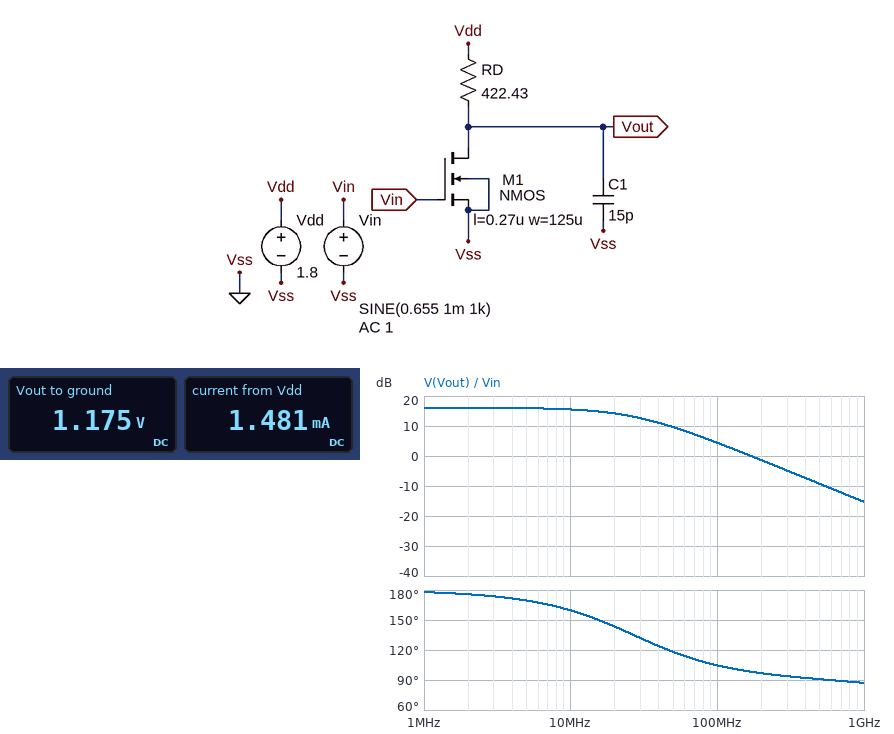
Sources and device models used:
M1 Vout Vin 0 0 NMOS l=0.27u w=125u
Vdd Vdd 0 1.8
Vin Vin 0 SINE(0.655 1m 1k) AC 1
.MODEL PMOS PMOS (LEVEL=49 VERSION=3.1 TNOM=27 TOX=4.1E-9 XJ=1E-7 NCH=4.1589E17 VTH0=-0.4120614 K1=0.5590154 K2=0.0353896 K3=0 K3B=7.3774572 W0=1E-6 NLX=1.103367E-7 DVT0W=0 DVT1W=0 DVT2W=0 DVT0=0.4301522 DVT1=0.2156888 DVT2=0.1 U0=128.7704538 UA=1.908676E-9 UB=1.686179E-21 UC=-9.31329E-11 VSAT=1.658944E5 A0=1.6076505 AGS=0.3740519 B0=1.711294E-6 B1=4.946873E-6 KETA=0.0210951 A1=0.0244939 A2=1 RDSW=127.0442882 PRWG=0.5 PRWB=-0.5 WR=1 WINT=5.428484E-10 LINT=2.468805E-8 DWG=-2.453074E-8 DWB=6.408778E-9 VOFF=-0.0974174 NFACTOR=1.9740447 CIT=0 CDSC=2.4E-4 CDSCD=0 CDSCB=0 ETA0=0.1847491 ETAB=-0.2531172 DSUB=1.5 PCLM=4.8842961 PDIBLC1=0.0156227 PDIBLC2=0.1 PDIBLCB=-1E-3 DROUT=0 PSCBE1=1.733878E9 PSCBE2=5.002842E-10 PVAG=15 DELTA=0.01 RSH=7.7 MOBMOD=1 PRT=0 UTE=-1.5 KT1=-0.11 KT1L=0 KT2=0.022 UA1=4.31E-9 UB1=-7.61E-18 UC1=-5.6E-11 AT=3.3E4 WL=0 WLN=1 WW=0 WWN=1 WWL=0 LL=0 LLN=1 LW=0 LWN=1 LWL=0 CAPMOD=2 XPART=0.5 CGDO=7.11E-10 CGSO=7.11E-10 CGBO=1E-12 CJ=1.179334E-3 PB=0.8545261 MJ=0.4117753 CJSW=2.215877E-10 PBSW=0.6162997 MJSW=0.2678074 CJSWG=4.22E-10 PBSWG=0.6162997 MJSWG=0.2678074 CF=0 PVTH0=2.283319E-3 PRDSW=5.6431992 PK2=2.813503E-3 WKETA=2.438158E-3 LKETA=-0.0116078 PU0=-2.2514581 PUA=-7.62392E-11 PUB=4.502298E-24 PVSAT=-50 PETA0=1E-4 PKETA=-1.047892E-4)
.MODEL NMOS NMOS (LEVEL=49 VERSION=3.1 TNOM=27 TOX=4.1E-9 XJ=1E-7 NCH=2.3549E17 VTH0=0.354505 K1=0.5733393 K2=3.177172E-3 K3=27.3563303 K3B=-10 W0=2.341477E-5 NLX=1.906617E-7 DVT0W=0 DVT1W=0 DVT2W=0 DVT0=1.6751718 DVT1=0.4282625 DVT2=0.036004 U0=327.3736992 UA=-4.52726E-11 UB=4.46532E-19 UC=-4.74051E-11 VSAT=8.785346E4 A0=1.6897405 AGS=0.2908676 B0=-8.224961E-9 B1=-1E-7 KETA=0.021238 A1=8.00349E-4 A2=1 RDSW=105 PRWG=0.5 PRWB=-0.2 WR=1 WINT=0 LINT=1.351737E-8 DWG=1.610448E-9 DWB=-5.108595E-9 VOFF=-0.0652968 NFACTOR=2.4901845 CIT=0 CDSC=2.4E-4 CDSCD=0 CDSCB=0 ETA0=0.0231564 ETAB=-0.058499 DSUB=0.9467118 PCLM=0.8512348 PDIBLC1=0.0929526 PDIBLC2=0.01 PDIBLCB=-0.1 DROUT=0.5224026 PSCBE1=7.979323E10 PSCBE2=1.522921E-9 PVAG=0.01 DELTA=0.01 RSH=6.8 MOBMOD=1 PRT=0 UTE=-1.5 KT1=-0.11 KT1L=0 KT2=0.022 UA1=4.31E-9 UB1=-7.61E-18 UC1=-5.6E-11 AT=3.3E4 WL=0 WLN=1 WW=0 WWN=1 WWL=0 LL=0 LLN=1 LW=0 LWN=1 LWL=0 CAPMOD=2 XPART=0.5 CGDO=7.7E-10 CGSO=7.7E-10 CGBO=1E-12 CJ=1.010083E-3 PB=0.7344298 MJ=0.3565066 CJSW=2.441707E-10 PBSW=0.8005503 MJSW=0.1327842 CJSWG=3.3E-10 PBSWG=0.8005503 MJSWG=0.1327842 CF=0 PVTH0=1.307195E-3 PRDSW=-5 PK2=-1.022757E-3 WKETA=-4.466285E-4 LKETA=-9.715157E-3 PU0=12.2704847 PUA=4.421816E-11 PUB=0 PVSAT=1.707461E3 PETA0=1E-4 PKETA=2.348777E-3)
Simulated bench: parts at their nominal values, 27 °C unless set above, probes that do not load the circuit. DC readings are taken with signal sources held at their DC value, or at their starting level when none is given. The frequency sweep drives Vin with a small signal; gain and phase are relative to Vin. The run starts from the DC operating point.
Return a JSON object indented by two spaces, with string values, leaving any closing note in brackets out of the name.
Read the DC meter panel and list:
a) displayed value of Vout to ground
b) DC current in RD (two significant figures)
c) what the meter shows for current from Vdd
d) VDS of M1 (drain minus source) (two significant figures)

{
  "displayed value of Vout to ground": "1.175 V",
  "DC current in RD": "1.5 mA",
  "what the meter shows for current from Vdd": "1.481 mA",
  "VDS of M1 (drain minus source)": "1.2 V"
}
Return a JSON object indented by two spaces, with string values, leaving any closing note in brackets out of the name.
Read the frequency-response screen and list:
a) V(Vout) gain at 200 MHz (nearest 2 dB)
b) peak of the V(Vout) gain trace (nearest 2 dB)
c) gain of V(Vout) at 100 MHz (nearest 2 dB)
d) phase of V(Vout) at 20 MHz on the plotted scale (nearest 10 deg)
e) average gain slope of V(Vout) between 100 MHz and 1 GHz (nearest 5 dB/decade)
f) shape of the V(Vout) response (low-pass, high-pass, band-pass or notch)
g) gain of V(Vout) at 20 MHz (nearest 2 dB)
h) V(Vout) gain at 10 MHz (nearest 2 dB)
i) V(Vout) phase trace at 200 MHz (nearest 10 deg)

{
  "V(Vout) gain at 200 MHz": "-2 dB",
  "peak of the V(Vout) gain trace": "16 dB",
  "gain of V(Vout) at 100 MHz": "4 dB",
  "phase of V(Vout) at 20 MHz on the plotted scale": "140 deg",
  "average gain slope of V(Vout) between 100 MHz and 1 GHz": "-20 dB/decade",
  "shape of the V(Vout) response": "low-pass",
  "gain of V(Vout) at 20 MHz": "14 dB",
  "V(Vout) gain at 10 MHz": "16 dB",
  "V(Vout) phase trace at 200 MHz": "100 deg"
}
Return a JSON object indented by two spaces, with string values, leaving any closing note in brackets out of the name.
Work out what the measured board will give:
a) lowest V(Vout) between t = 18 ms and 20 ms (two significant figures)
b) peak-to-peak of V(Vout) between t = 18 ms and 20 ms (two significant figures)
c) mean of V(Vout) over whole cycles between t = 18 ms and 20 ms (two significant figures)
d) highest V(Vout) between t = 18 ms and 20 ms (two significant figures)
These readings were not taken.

{
  "lowest V(Vout) between t = 18 ms and 20 ms": "1.2 V",
  "peak-to-peak of V(Vout) between t = 18 ms and 20 ms": "13 mV",
  "mean of V(Vout) over whole cycles between t = 18 ms and 20 ms": "1.2 V",
  "highest V(Vout) between t = 18 ms and 20 ms": "1.2 V"
}
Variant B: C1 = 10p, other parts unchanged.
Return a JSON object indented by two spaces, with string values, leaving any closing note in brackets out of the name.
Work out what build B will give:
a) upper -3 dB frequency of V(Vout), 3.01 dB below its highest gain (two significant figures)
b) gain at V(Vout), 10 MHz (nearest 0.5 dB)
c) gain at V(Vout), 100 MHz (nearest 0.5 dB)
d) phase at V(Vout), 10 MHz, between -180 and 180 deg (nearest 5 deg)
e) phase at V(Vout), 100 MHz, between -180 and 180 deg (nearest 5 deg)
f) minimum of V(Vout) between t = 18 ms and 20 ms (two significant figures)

{
  "upper -3 dB frequency of V(Vout), 3.01 dB below its highest gain": "40 MHz",
  "gain at V(Vout), 10 MHz": "16.0 dB",
  "gain at V(Vout), 100 MHz": "7.5 dB",
  "phase at V(Vout), 10 MHz, between -180 and 180 deg": "165 deg",
  "phase at V(Vout), 100 MHz, between -180 and 180 deg": "110 deg",
  "minimum of V(Vout) between t = 18 ms and 20 ms": "1.2 V"
}
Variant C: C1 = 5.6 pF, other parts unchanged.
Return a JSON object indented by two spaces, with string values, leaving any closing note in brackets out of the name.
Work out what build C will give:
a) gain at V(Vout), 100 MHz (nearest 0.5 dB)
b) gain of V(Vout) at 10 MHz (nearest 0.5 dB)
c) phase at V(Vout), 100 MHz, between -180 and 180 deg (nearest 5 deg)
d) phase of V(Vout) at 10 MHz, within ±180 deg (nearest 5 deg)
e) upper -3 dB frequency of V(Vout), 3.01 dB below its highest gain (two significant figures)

{
  "gain at V(Vout), 100 MHz": "11.5 dB",
  "gain of V(Vout) at 10 MHz": "16.0 dB",
  "phase at V(Vout), 100 MHz, between -180 and 180 deg": "125 deg",
  "phase of V(Vout) at 10 MHz, within ±180 deg": "170 deg",
  "upper -3 dB frequency of V(Vout), 3.01 dB below its highest gain": "71 MHz"
}
